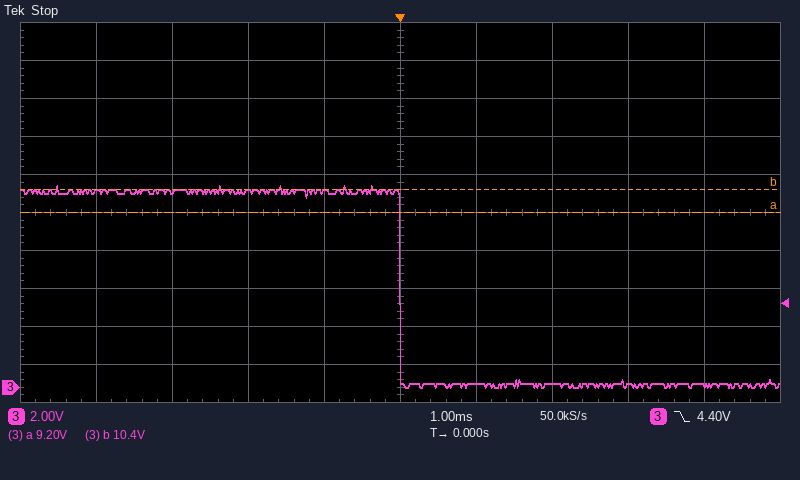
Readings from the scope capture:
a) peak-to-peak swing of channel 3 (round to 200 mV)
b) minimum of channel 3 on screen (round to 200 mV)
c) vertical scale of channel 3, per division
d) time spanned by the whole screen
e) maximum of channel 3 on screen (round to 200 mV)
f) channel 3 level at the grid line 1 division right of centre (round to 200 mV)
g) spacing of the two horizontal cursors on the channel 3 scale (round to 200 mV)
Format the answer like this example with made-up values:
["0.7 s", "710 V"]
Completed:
["10.6 V", "0.0 V", "2 V", "10 ms", "10.6 V", "200 mV", "1.2 V"]
